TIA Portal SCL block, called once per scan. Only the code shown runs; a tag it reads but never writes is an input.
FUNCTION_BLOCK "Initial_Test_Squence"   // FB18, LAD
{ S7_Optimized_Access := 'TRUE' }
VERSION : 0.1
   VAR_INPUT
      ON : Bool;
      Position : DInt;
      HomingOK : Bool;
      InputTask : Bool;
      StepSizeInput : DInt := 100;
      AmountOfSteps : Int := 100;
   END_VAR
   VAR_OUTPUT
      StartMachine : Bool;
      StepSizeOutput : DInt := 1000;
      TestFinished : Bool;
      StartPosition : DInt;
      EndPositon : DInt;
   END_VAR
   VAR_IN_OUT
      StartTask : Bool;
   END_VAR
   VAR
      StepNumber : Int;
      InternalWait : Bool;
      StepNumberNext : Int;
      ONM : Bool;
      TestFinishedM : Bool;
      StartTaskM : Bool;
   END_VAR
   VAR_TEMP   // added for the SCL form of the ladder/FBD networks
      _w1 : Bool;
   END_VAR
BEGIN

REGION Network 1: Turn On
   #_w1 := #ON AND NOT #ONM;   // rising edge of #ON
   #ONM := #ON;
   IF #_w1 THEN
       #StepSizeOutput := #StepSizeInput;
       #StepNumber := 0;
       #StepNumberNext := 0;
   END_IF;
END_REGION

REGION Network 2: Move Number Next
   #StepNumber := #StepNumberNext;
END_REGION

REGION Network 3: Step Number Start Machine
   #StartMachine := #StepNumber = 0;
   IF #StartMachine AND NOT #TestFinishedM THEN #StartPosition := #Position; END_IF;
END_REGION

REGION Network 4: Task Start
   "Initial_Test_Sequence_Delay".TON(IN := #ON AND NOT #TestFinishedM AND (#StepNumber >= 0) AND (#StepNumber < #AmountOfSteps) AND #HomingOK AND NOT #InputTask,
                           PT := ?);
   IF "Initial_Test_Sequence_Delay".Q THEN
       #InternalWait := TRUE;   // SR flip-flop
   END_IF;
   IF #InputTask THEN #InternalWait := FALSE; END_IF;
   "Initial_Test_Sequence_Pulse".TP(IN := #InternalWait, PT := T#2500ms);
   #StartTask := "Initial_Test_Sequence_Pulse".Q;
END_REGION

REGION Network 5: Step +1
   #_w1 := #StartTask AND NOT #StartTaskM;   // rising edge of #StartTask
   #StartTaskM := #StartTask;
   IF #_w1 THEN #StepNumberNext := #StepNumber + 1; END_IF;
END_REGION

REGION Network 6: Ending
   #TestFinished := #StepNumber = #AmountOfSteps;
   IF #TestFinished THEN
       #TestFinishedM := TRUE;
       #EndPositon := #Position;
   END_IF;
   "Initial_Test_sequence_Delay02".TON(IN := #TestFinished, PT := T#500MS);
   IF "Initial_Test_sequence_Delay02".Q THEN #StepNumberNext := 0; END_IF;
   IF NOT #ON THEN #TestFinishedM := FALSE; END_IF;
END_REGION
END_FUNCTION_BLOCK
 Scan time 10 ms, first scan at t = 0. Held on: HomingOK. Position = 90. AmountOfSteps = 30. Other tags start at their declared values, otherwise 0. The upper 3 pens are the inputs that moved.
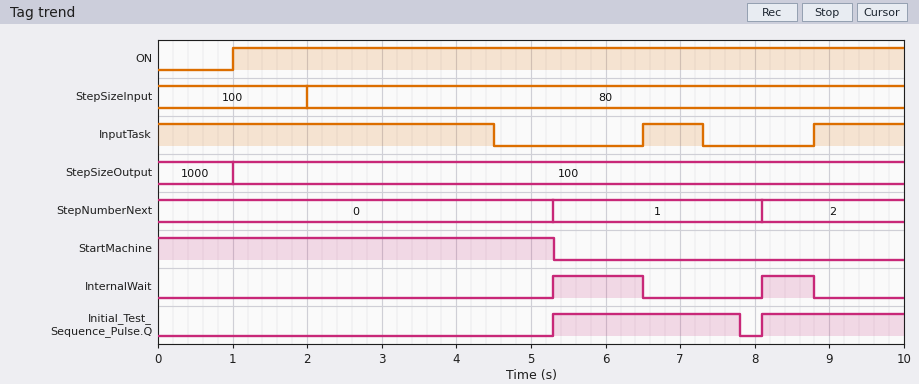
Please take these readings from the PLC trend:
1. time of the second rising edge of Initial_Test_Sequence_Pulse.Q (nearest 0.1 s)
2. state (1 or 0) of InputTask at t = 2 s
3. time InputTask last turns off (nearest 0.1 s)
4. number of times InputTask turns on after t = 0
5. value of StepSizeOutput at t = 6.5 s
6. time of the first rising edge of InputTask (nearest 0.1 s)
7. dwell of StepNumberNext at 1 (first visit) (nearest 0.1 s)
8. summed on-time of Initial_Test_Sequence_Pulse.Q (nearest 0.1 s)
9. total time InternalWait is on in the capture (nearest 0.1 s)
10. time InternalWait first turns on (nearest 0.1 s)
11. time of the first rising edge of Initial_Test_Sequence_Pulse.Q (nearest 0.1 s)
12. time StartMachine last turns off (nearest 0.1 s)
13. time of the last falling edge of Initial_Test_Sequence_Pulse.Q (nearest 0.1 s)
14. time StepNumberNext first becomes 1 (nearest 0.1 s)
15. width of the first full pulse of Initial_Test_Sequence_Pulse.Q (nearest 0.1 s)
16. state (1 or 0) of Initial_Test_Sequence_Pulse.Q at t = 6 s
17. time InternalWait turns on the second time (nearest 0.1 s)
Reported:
8.1 s
1
7.3 s
2
100
6.5 s
2.8 s
4.4 s
1.9 s
5.3 s
5.3 s
5.3 s
7.8 s
5.3 s
2.5 s
1
8.1 s
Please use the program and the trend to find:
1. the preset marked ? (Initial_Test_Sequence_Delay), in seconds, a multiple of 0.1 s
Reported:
0.8 s
